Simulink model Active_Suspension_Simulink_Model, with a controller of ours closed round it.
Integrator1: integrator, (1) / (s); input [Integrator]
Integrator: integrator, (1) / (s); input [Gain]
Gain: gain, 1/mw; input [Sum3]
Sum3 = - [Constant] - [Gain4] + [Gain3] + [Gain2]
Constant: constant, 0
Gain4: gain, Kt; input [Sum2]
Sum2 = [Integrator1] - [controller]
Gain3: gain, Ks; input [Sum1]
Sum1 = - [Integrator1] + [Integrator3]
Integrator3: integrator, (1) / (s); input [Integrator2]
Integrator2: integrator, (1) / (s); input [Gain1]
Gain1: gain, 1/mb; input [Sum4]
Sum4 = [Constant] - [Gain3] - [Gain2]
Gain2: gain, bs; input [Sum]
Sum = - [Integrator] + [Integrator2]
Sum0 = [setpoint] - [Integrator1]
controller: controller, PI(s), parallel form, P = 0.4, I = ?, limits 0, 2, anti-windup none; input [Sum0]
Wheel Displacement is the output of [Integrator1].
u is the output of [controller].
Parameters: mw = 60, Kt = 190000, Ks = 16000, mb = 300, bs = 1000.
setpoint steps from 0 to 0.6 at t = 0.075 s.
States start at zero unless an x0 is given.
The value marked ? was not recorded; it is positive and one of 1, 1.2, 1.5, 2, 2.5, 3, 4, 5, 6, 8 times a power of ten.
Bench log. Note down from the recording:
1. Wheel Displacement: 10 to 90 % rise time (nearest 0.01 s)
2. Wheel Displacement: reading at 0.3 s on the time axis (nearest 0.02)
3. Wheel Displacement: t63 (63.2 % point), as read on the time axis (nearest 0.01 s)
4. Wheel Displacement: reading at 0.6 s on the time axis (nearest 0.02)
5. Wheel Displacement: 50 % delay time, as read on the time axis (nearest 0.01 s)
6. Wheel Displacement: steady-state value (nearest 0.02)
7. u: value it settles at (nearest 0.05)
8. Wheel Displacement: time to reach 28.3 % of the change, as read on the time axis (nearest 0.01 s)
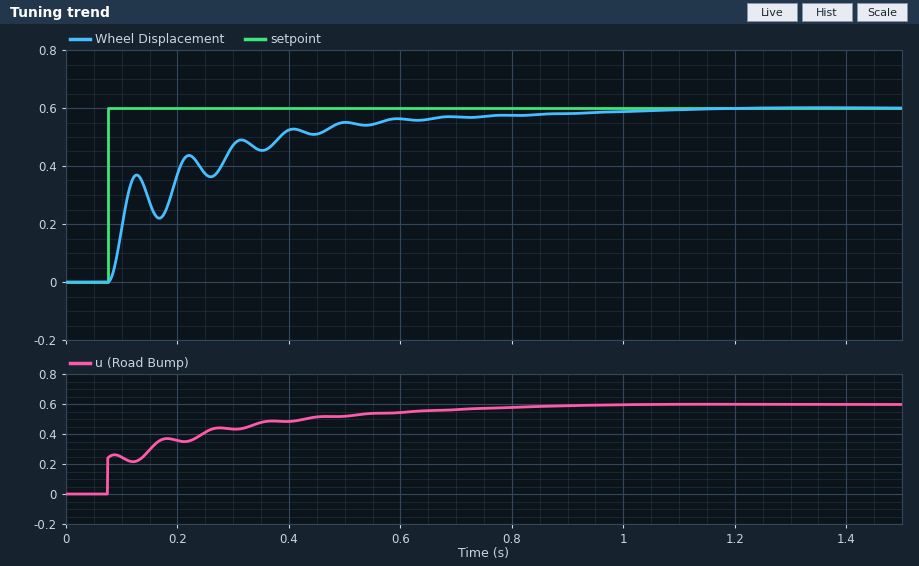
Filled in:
0.39 s
0.48
0.20 s
0.56
0.11 s
0.60
0.60
0.10 s
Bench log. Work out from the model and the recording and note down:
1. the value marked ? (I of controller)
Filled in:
6
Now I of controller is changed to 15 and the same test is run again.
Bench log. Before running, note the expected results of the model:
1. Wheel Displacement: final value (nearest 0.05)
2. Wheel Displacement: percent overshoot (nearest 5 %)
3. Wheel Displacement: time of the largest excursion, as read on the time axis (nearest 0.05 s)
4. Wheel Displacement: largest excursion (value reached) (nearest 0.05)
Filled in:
0.60
10 %
0.30 s
0.65
